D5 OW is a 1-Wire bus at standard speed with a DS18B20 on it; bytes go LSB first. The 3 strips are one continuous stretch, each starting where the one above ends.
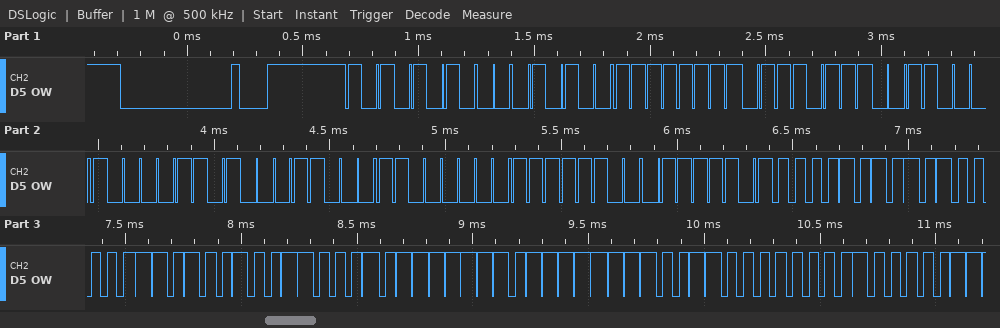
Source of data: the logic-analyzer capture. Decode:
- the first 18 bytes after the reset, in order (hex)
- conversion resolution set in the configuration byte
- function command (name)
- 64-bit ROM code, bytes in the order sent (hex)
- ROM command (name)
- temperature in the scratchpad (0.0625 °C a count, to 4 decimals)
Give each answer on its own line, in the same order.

55 28 FF EE 8C B0 18 03 3F BE 50 05 4B 46 7F FF 0C 10
12 bits
Read Scratchpad
28 FF EE 8C B0 18 03 3F
Match ROM
85.0000 °C
